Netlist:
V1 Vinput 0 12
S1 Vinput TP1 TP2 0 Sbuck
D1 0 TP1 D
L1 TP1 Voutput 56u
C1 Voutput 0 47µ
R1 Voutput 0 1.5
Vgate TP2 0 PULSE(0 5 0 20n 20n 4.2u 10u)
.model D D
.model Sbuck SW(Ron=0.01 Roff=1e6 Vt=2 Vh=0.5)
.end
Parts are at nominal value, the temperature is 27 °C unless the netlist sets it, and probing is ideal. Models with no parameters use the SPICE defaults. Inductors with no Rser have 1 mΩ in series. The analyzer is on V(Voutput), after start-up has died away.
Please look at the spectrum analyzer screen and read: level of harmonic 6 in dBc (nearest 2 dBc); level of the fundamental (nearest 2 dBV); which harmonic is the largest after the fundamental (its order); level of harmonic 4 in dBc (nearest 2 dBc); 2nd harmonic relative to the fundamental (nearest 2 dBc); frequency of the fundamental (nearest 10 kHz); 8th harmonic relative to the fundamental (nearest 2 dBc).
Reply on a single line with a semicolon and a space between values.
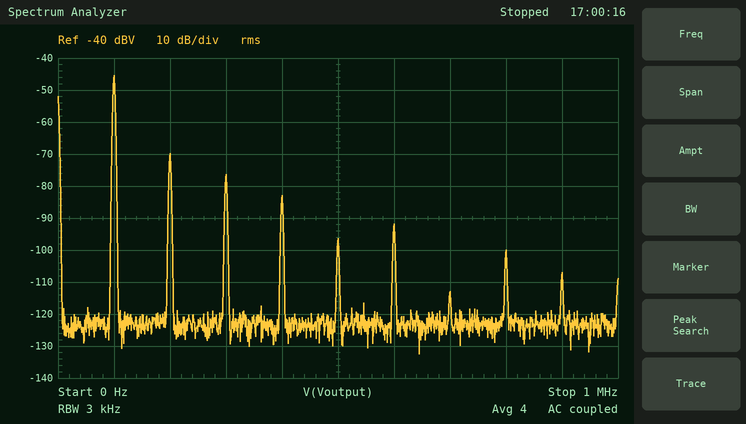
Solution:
-46 dBc; -46 dBV; 2; -38 dBc; -24 dBc; 100 kHz; -54 dBc
